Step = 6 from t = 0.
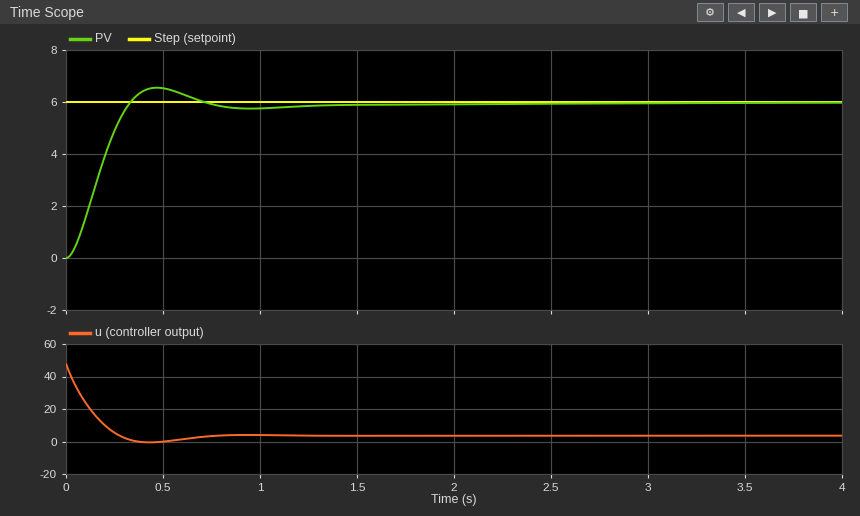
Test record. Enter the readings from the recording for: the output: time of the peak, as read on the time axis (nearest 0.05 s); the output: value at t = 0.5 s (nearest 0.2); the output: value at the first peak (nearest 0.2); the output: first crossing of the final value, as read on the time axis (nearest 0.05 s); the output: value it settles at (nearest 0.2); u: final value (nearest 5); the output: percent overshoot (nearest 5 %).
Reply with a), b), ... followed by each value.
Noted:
a) 0.45 s
b) 6.6
c) 6.6
d) 0.35 s
e) 6.0
f) 5
g) 10 %
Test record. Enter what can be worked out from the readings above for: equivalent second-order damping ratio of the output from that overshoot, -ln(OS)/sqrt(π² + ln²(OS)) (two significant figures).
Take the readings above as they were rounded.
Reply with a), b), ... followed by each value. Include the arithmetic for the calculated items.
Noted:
a) ln(0.1) = -2.303; 2.303 / sqrt(9.870 + 5.302) = 0.59
